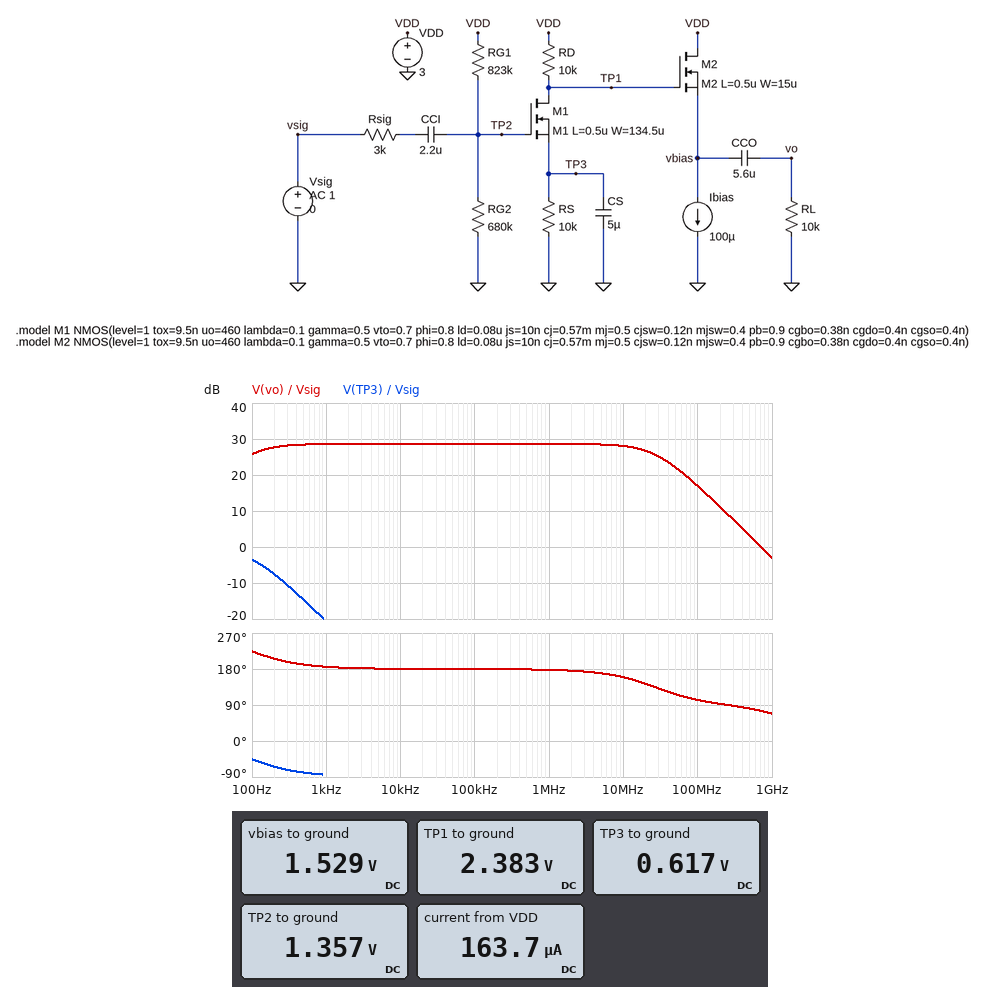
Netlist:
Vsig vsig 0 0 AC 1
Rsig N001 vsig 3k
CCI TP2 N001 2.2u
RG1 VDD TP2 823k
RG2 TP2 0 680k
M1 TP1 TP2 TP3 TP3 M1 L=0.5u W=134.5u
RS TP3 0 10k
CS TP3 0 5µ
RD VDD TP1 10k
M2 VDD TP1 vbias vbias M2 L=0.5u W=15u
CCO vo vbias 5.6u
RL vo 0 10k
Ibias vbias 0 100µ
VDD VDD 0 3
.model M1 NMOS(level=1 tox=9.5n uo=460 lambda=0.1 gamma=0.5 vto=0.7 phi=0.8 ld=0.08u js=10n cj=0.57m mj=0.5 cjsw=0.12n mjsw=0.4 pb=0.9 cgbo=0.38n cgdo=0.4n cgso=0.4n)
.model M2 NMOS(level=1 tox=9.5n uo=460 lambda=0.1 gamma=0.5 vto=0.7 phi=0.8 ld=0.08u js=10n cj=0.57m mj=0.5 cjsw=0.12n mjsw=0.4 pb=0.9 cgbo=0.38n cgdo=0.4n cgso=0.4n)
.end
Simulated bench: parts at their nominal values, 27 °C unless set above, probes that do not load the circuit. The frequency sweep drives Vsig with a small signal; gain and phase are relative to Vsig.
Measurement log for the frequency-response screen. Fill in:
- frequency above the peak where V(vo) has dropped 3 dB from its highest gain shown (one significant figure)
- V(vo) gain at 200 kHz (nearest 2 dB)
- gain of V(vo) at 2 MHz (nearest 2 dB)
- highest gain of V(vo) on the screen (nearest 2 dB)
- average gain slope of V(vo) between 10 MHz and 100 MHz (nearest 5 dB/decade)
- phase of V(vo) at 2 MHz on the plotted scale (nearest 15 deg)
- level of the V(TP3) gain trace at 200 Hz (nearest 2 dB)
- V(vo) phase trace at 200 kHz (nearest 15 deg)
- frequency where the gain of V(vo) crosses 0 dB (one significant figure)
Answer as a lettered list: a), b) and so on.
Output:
a) 30 MHz
b) 28 dB
c) 28 dB
d) 28 dB
e) -10 dB/decade
f) 180 deg
g) -8 dB
h) 180 deg
i) 700 MHz
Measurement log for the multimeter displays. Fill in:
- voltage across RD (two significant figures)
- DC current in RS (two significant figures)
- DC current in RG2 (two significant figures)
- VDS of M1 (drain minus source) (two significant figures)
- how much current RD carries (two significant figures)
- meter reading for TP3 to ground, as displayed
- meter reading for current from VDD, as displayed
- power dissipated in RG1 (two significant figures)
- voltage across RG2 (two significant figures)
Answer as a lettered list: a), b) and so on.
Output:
a) 620 mV
b) 62 µA
c) 2.0 µA
d) 1.8 V
e) 62 µA
f) 0.617 V
g) 163.7 µA
h) 3.3 µW
i) 1.4 V
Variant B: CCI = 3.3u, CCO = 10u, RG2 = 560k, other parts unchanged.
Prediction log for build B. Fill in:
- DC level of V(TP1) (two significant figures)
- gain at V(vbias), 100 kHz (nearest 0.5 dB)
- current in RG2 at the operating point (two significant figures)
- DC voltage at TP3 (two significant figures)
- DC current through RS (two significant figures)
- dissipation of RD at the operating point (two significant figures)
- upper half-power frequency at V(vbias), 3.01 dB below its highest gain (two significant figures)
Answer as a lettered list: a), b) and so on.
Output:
a) 2.5 V
b) 27.5 dB
c) 2.2 µA
d) 480 mV
e) 48 µA
f) 23 µW
g) 29 MHz
